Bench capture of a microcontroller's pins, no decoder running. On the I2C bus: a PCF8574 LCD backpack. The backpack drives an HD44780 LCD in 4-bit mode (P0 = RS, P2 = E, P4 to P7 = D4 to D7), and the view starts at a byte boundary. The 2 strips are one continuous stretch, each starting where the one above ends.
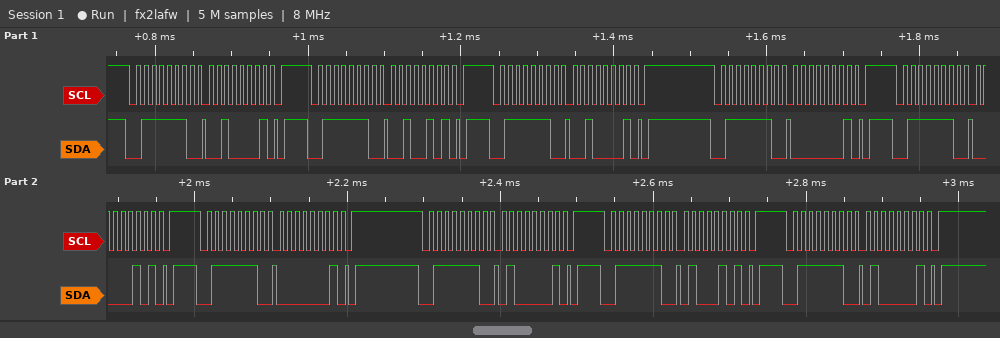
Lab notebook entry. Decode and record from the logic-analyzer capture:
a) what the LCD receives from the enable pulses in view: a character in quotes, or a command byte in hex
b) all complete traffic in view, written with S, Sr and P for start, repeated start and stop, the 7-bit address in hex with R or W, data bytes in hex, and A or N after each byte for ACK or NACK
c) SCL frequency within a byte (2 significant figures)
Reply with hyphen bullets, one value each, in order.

- ' '
- S 3FW A 21 A P S 3FW A 25 A P S 3FW A 21 A P S 3FW A 01 A P S 3FW A 05 A P S 3FW A 01 A P S 3FW A 41 A P S 3FW A 45 A P S 3FW A 41 A P
- 100 kHz
